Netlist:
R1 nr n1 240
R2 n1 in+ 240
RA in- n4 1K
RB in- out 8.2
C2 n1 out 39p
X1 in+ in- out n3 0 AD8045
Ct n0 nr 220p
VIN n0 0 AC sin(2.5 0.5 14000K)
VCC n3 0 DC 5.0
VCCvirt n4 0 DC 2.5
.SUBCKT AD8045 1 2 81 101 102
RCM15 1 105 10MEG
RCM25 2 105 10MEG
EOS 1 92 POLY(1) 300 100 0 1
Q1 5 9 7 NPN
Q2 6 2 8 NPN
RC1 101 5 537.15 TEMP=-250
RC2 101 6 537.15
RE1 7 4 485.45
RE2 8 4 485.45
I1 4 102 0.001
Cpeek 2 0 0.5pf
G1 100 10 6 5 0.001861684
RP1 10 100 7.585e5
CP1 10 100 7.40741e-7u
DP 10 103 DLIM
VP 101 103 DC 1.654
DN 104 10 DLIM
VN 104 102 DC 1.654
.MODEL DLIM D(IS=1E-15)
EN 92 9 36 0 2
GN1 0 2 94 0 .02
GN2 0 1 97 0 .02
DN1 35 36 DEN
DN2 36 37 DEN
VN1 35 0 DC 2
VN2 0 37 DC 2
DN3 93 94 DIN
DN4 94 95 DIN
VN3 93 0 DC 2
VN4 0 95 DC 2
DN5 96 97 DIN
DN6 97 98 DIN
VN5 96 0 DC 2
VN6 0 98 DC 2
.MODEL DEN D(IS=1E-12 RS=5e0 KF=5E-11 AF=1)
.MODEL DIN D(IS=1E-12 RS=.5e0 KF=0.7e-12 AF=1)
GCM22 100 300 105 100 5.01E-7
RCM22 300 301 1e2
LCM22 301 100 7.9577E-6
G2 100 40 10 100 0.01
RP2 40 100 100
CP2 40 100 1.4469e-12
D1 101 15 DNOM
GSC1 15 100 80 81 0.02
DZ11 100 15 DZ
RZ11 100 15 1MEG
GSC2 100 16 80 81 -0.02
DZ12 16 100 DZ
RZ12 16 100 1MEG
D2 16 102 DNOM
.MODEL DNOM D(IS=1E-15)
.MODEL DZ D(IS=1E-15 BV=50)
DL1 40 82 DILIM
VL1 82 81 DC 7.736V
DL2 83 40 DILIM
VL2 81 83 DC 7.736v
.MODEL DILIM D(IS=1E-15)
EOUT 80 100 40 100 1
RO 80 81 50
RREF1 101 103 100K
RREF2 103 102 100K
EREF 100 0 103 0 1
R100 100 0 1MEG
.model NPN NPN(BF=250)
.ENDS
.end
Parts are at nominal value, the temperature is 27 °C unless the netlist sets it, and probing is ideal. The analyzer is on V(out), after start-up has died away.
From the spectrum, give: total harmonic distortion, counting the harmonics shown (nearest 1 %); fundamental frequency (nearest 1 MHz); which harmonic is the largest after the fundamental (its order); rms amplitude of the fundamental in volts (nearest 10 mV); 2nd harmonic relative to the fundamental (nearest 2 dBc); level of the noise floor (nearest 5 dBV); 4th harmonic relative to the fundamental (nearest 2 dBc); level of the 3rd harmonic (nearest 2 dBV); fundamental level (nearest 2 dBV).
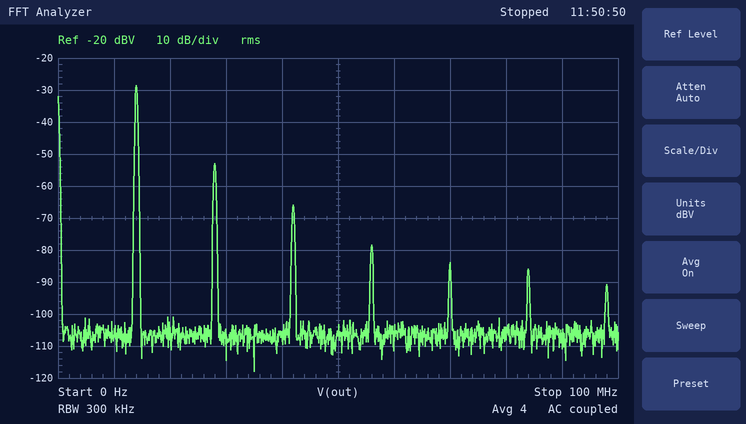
6 %
14 MHz
2
40 mV
-24 dBc
-105 dBV
-50 dBc
-66 dBV
-28 dBV
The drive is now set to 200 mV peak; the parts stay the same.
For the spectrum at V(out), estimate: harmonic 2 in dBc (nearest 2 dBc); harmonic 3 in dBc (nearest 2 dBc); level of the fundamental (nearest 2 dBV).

-30 dBc
-46 dBc
-36 dBV
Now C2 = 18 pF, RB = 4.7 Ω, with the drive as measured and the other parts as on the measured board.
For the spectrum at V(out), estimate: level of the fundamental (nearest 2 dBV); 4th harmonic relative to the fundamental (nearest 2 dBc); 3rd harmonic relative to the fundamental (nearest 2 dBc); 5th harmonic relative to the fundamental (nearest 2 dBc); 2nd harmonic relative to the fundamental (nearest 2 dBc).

-32 dBV
-48 dBc
-28 dBc
-50 dBc
-16 dBc
